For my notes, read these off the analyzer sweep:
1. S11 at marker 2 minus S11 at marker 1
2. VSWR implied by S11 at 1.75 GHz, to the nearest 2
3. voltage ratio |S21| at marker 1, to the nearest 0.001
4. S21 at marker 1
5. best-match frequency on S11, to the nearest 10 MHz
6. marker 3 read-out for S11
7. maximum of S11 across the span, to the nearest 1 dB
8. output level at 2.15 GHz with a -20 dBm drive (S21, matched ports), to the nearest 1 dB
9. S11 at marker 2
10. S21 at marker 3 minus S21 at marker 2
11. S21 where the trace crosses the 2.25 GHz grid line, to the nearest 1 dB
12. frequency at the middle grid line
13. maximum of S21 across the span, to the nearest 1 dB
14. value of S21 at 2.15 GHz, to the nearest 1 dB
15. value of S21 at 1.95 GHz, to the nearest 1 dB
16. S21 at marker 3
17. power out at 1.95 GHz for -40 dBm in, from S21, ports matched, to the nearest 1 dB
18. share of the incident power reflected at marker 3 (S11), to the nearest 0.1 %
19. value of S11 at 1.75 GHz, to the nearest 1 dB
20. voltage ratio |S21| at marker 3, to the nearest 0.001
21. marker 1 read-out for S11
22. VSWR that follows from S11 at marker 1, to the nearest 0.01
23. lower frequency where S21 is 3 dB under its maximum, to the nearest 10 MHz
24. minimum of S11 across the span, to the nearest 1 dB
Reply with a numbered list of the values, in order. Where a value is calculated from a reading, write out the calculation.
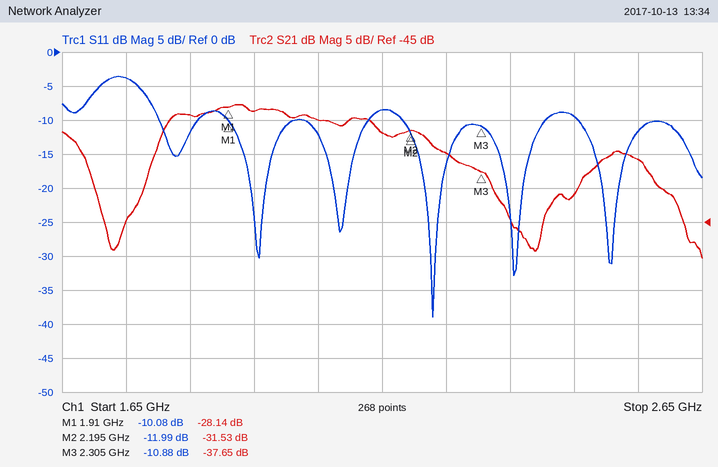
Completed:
1. -11.99 − (-10.08) = -1.91 dB
2. |Γ| = 10^(-4/20) = 0.6310; VSWR = (1 + 0.6310)/(1 − 0.6310) ≈ 4
3. 10^(-28.14/20) ≈ 0.039
4. -28.14 dB
5. 2.23 GHz
6. -10.88 dB
7. -4 dB
8. -20 dBm + (-32 dB) = -52 dBm
9. -11.99 dB
10. -37.65 − (-31.53) = -6.12 dB
11. -35 dB
12. 2.15 GHz
13. -28 dB
14. -32 dB
15. -29 dB
16. -37.65 dB
17. -40 dBm + (-29 dB) = -69 dBm
18. 10^(-10.88/10) ≈ 8.2 %
19. -4 dB
20. 10^(-37.65/20) ≈ 0.013
21. -10.08 dB
22. (1 + 0.3133)/(1 − 0.3133) ≈ 1.91
23. 1.81 GHz
24. -39 dB
